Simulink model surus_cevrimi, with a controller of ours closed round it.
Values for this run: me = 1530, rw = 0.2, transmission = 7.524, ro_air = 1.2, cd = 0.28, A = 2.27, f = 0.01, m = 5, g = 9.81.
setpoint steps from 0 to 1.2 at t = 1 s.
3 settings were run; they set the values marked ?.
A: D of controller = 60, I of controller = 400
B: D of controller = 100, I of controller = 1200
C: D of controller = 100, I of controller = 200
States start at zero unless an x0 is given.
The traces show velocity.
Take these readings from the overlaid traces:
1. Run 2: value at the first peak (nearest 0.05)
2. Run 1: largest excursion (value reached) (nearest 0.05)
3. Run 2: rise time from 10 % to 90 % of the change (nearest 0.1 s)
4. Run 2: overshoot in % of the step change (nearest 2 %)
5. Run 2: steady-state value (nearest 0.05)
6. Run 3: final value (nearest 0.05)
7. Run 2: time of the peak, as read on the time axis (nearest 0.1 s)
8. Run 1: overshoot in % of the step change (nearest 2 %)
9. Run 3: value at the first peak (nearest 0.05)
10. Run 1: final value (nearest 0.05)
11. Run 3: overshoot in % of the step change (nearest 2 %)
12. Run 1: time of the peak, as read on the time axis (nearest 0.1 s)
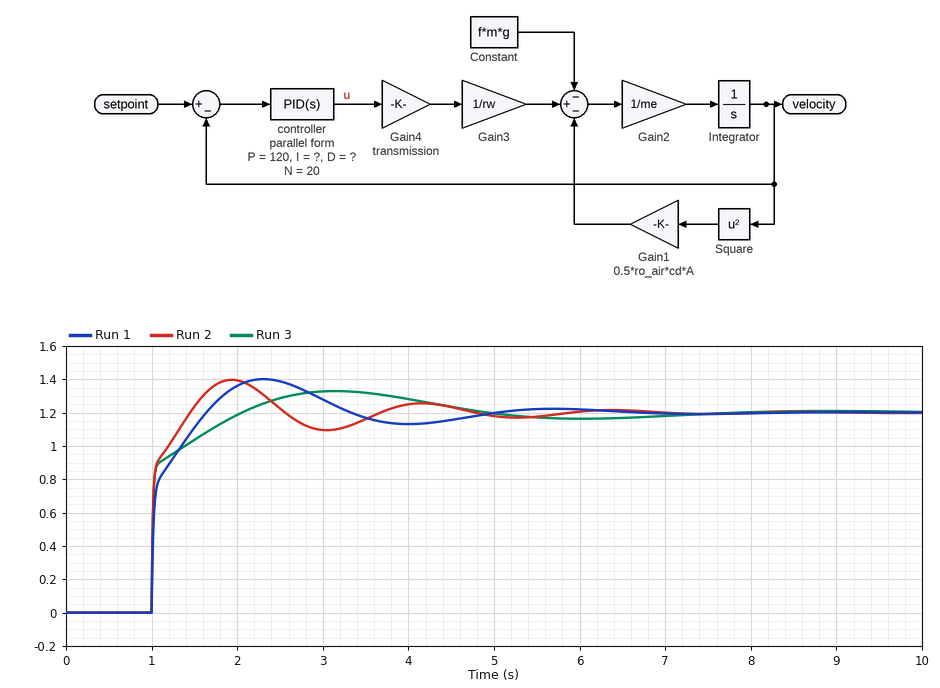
1.40
1.40
0.3 s
16 %
1.20
1.20
1.9 s
16 %
1.35
1.20
10 %
2.3 s
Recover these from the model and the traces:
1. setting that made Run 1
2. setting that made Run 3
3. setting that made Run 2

A
C
B
